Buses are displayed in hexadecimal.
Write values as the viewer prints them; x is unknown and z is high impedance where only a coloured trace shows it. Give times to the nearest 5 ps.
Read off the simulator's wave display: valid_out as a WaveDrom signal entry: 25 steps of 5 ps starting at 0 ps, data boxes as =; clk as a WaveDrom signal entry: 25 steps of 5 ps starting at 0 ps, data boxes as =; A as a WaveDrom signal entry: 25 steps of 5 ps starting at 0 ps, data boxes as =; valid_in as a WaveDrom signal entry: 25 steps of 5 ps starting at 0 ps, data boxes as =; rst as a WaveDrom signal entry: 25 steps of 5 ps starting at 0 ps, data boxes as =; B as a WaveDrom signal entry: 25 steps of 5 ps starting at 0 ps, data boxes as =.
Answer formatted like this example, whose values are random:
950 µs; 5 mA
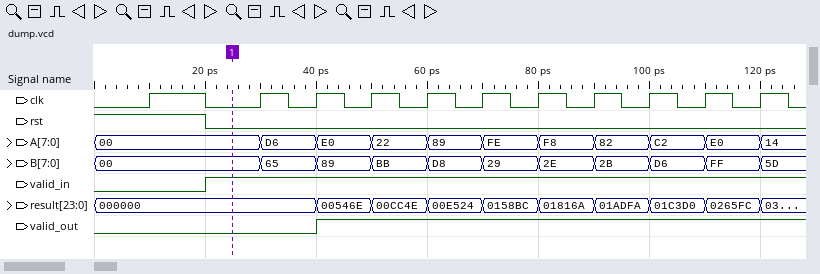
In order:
{name: 'valid_out', wave: '0.......1................'}; {name: 'clk', wave: '0.1.0.1010101010101010101'}; {name: 'A', wave: '=.....=.=.=.=.=.=.=.=.=.=', data: '00 D6 E0 22 89 FE F8 82 C2 E0 14'}; {name: 'valid_in', wave: '0...1....................'}; {name: 'rst', wave: '1...0....................'}; {name: 'B', wave: '=.....=.=.=.=.=.=.=.=.=.=', data: '00 65 89 BB D8 29 2E 2B D6 FF 5D'}
